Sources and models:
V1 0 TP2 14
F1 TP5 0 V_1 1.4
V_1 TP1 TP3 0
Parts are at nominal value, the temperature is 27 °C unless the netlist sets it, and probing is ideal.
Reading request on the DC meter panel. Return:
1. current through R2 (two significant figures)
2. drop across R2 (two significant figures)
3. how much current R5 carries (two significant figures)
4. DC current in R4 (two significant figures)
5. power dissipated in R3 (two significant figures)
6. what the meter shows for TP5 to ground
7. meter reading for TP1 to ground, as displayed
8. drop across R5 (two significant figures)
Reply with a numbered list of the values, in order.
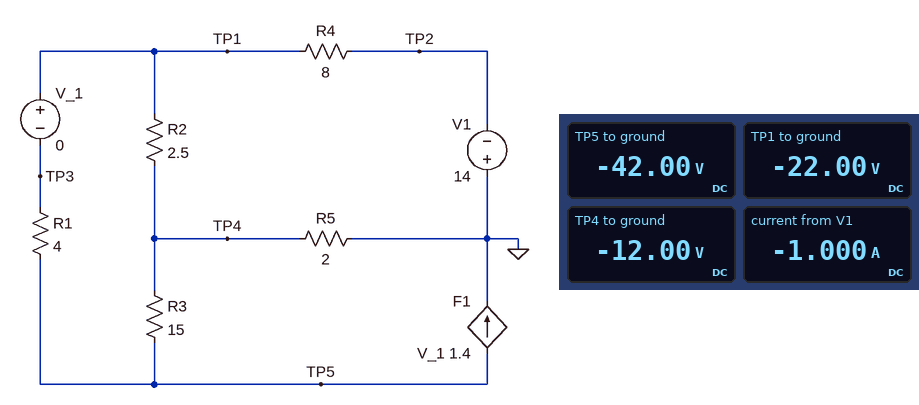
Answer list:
1. 4.0 A
2. 10 V
3. 6.0 A
4. 1.0 A
5. 60 W
6. -42.00 V
7. -22.00 V
8. 12 V
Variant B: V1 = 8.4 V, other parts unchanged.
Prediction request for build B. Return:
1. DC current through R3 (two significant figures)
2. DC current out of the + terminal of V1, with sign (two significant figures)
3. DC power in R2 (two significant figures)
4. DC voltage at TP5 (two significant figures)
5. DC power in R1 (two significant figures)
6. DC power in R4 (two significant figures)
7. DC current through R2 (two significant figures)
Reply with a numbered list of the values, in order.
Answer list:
1. 1.2 A
2. -600 mA
3. 14 W
4. -25 V
5. 36 W
6. 2.9 W
7. 2.4 A
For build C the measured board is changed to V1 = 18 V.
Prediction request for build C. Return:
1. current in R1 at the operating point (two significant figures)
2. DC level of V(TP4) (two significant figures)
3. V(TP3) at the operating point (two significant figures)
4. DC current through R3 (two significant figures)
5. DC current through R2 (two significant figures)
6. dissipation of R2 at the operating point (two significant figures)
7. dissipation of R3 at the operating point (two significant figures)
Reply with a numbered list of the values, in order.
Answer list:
1. 6.4 A
2. -15 V
3. -28 V
4. 2.6 A
5. 5.1 A
6. 66 W
7. 99 W
